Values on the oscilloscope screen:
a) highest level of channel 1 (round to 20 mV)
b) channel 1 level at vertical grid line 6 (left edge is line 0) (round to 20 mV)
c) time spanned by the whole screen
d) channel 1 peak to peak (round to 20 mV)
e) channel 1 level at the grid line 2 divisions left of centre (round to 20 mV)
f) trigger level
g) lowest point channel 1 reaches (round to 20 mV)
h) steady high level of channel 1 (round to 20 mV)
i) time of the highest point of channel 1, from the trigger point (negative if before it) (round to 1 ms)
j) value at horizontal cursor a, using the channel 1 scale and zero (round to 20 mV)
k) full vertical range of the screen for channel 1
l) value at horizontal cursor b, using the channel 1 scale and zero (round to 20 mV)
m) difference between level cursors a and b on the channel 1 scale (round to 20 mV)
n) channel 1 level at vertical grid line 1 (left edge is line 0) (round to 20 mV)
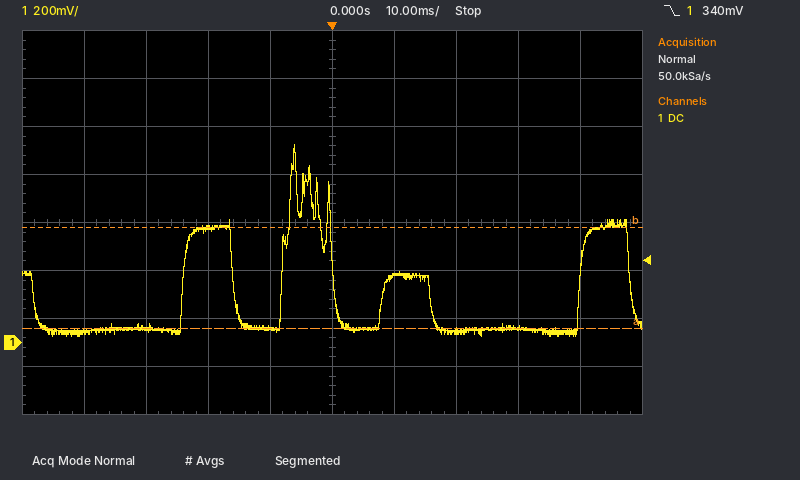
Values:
820 mV
280 mV
100 ms
800 mV
480 mV
340 mV
20 mV
480 mV
-6 ms
60 mV
1.6 V
480 mV
420 mV
40 mV
